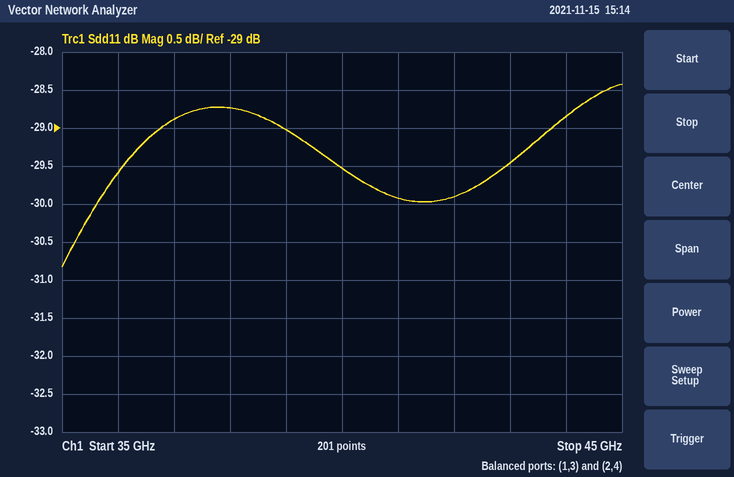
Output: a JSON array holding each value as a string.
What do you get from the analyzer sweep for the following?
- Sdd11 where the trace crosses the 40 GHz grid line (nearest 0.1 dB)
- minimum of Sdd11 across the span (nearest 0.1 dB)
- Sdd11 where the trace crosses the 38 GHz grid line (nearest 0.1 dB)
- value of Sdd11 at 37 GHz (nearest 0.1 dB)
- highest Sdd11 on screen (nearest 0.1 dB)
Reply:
["-29.5 dB", "-30.8 dB", "-28.7 dB", "-28.9 dB", "-28.4 dB"]
